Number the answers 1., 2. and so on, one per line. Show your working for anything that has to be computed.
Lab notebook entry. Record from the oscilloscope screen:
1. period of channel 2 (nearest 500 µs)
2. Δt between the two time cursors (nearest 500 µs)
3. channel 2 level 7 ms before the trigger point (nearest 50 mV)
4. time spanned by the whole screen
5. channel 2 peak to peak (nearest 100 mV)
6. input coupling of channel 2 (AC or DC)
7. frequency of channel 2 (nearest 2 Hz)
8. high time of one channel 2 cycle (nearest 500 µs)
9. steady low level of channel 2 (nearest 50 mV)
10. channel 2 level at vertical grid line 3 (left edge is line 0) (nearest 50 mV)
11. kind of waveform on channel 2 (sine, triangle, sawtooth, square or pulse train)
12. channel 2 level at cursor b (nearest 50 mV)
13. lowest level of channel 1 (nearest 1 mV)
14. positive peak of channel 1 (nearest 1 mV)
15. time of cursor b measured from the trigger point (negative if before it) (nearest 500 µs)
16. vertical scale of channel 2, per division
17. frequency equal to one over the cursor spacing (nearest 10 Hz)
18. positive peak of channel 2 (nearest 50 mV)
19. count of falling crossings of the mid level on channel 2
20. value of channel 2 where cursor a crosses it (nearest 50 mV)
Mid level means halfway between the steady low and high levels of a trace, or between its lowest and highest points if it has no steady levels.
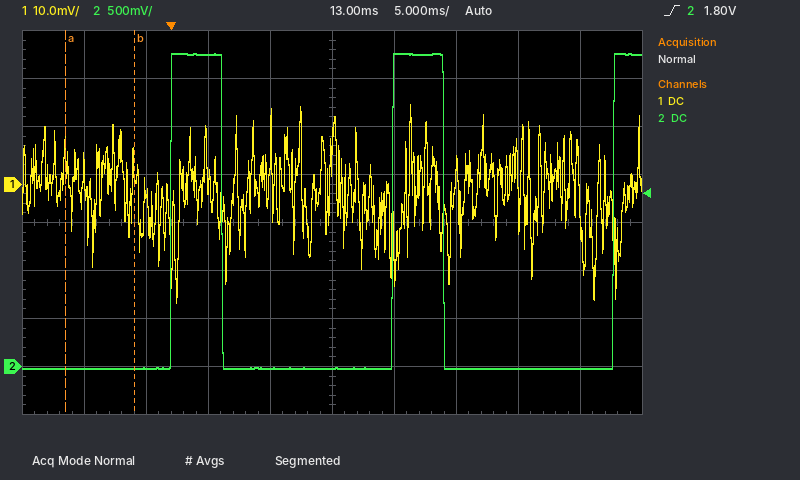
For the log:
1. 18.0 ms
2. 5.5 ms
3. 0 mV
4. 50 ms
5. 3.30 V
6. DC
7. 1 / 18.0 ms ≈ 56 Hz
8. 4.0 ms
9. 0 mV
10. 3.25 V
11. pulse train
12. 0 mV
13. -25 mV
14. 17 mV
15. -3.0 ms
16. 500 mV
17. 1 / 5.5 ms ≈ 180 Hz
18. 3.25 V
19. 2
20. 0 mV
